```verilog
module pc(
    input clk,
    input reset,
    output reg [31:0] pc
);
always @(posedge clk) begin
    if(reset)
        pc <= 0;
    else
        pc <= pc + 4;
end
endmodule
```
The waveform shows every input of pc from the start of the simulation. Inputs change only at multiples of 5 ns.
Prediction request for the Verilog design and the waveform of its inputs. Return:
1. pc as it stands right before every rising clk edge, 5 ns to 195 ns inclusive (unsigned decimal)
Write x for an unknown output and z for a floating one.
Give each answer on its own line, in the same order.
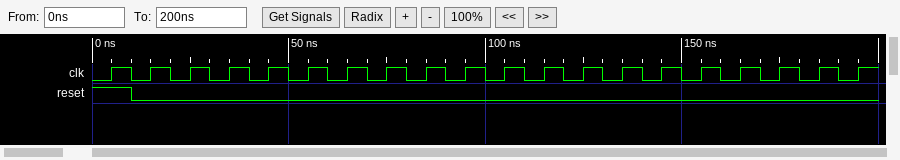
x, 0, 4, 8, 12, 16, 20, 24, 28, 32, 36, 40, 44, 48, 52, 56, 60, 64, 68, 72
